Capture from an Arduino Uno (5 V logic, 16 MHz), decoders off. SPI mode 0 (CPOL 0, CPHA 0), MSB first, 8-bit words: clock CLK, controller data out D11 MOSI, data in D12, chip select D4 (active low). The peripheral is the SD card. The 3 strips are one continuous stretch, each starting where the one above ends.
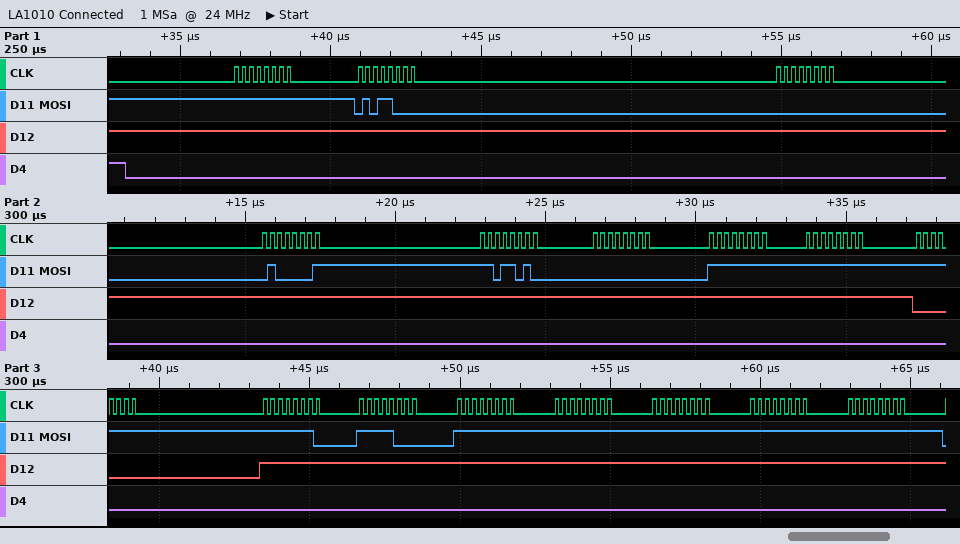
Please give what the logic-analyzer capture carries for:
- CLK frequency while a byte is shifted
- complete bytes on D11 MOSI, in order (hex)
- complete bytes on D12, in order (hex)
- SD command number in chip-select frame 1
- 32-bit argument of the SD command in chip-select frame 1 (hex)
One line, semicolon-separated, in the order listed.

4 MHz; FF 58 00 41 DA 00 FF FF FF FE F8 FF FF FF FF FF; FF FF FF FF FF FF FF FF 00 FF FF FF FF FF FF FF; CMD24; 0x0041DA00
